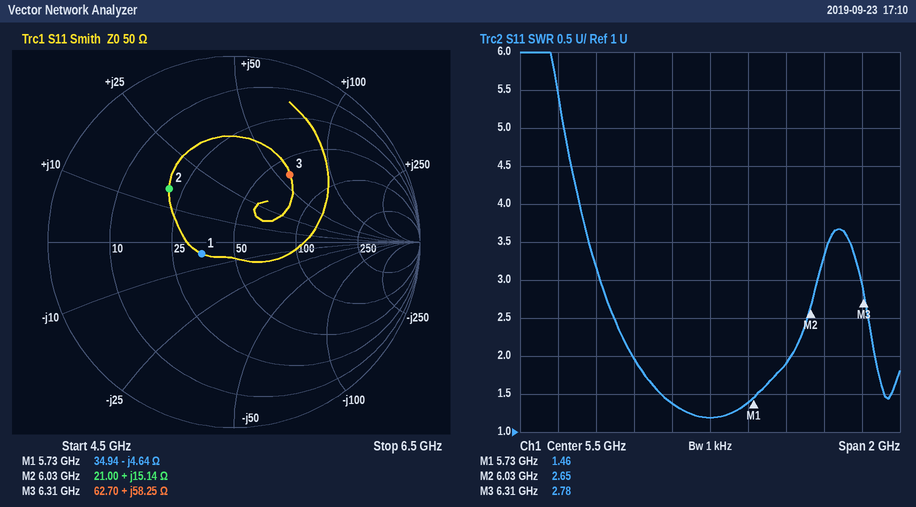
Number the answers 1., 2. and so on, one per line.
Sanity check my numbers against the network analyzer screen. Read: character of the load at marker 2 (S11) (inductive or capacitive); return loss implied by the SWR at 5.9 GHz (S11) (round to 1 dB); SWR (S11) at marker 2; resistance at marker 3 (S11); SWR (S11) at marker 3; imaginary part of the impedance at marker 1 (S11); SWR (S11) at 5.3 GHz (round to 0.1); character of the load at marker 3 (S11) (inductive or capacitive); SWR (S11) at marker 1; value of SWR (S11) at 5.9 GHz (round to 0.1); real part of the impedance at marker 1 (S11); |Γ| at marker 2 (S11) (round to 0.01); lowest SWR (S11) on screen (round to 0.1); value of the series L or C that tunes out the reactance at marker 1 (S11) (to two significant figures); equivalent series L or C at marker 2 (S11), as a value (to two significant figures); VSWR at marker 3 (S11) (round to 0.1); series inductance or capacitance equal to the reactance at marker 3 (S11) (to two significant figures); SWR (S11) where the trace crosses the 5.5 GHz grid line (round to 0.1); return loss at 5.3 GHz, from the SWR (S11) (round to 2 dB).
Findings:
1. inductive
2. 10 dB
3. 2.65
4. 62.70 Ω
5. 2.78
6. -4.64 Ω
7. 1.4
8. inductive
9. 1.46
10. 1.9
11. 34.94 Ω
12. 0.45
13. 1.2
14. 130 pH
15. 400 pH
16. 2.8
17. 1.5 nH
18. 1.2
19. 16 dB
